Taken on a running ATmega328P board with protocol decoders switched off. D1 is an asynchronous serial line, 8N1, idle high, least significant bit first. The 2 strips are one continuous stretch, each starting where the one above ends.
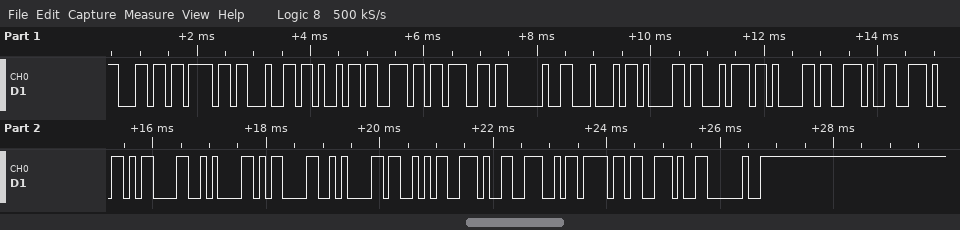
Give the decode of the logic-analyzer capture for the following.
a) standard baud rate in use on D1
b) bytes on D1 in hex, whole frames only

9600 baud
0x6C 0x6F 0x64 0x69 0x6E 0x67 0x20 0x44 0x61 0x74 0x61 0x2E 0x2E 0x0D 0x0A 0x0D 0x0A 0x53 0x2E 0x4E 0x6F 0x2E 0x20
